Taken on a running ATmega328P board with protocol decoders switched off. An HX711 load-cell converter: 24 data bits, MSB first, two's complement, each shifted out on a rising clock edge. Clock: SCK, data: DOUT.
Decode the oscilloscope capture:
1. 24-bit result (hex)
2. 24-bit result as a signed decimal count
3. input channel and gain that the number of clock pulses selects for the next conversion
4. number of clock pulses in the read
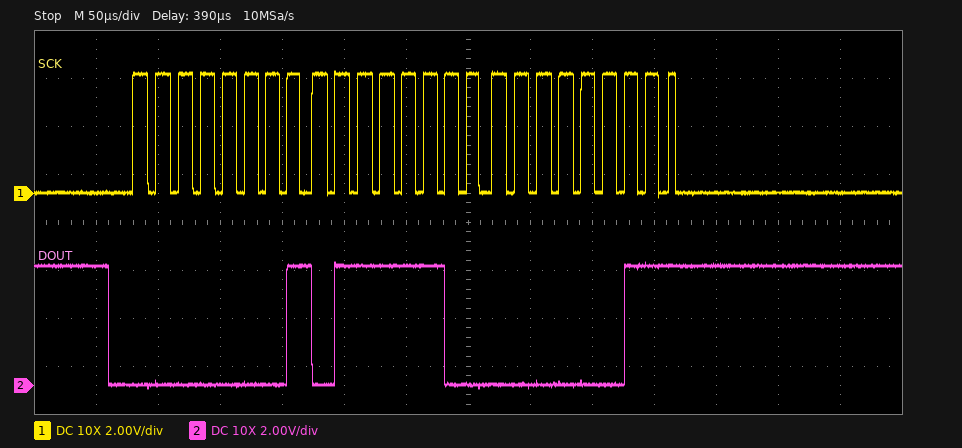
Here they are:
0x017C03
97283
channel A, gain 128
25
